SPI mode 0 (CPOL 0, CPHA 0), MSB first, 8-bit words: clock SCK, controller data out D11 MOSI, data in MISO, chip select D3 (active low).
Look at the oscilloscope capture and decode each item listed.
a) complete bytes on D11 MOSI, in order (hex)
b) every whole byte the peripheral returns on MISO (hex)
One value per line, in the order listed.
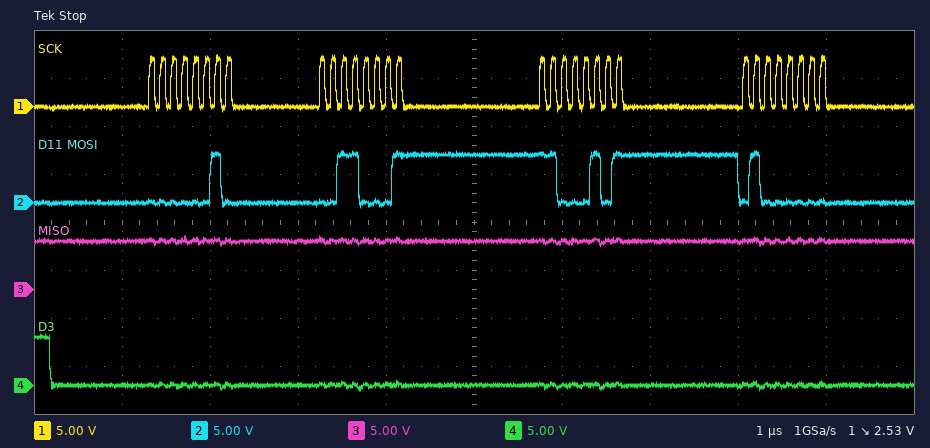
02 31 C5 40
FF FF FF FF
